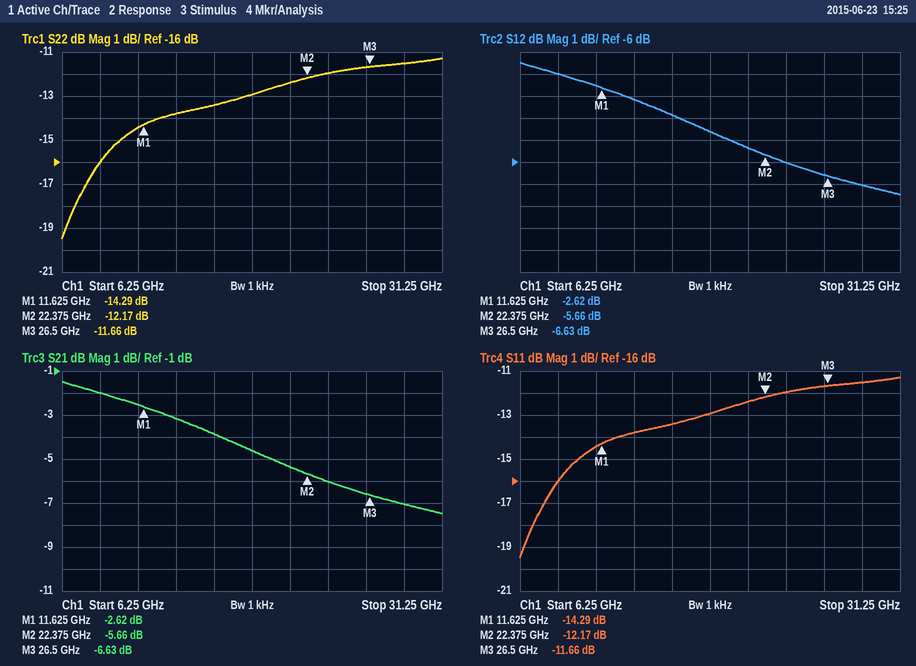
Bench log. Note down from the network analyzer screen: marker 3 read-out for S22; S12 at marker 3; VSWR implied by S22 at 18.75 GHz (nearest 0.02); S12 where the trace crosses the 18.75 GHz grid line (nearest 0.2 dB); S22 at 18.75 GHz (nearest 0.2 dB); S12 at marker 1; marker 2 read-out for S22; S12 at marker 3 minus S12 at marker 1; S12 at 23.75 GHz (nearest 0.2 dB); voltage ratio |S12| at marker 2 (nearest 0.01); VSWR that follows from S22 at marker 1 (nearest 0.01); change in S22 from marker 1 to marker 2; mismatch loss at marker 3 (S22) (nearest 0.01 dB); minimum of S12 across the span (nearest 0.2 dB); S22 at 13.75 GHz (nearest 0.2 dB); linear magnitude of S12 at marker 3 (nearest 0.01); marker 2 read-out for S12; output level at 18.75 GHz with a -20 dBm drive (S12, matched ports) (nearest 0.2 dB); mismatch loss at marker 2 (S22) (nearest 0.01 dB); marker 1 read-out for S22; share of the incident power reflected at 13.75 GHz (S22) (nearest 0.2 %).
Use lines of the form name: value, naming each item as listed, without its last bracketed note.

marker 3 read-out for S22: -11.66 dB
S12 at marker 3: -6.63 dB
VSWR implied by S22 at 18.75 GHz: 1.58
S12 where the trace crosses the 18.75 GHz grid line: -4.6 dB
S22 at 18.75 GHz: -13.0 dB
S12 at marker 1: -2.62 dB
marker 2 read-out for S22: -12.17 dB
S12 at marker 3 minus S12 at marker 1: -4.01 dB
S12 at 23.75 GHz: -6.0 dB
voltage ratio |S12| at marker 2: 0.52
VSWR that follows from S22 at marker 1: 1.48
change in S22 from marker 1 to marker 2: 2.12 dB
mismatch loss at marker 3 (S22): 0.31 dB
minimum of S12 across the span: -7.4 dB
S22 at 13.75 GHz: -13.8 dB
linear magnitude of S12 at marker 3: 0.47
marker 2 read-out for S12: -5.66 dB
output level at 18.75 GHz with a -20 dBm drive (S12, matched ports): -24.6 dBm
mismatch loss at marker 2 (S22): 0.27 dB
marker 1 read-out for S22: -14.29 dB
share of the incident power reflected at 13.75 GHz (S22): 4.2 %
